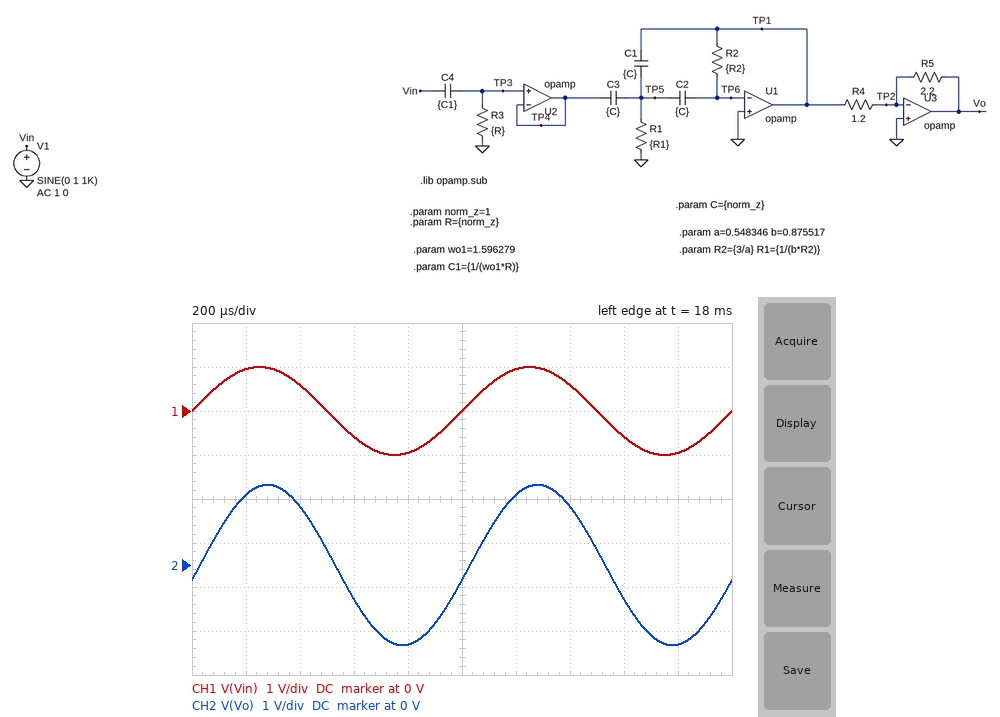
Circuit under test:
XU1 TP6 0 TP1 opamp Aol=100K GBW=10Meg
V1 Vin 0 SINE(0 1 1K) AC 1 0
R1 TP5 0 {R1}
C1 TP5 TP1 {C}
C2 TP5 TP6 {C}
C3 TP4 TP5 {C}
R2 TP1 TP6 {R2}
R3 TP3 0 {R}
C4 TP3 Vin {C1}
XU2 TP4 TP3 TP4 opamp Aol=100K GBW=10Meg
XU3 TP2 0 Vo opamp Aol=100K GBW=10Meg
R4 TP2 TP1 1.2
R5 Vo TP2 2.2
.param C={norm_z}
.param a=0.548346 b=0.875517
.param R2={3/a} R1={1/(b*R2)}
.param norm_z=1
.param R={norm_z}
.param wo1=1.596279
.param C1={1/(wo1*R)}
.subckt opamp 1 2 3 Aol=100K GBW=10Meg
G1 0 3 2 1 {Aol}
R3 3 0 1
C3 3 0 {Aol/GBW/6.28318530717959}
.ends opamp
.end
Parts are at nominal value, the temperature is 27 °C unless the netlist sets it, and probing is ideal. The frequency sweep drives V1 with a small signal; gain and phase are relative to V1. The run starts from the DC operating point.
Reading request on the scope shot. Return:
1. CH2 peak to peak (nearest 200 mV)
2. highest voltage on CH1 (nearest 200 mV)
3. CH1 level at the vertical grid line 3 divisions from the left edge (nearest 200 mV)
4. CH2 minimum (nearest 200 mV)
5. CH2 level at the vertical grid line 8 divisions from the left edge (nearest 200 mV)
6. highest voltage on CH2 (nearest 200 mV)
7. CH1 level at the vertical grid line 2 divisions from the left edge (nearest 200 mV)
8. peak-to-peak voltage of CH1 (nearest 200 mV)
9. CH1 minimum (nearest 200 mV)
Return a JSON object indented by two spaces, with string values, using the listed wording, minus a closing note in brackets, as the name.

{
  "CH2 peak to peak": "3.6 V",
  "highest voltage on CH1": "1.0 V",
  "CH1 level at the vertical grid line 3 divisions from the left edge": "-600 mV",
  "CH2 minimum": "-1.8 V",
  "CH2 level at the vertical grid line 8 divisions from the left edge": "-800 mV",
  "highest voltage on CH2": "1.8 V",
  "CH1 level at the vertical grid line 2 divisions from the left edge": "600 mV",
  "peak-to-peak voltage of CH1": "2.0 V",
  "CH1 minimum": "-1.0 V"
}
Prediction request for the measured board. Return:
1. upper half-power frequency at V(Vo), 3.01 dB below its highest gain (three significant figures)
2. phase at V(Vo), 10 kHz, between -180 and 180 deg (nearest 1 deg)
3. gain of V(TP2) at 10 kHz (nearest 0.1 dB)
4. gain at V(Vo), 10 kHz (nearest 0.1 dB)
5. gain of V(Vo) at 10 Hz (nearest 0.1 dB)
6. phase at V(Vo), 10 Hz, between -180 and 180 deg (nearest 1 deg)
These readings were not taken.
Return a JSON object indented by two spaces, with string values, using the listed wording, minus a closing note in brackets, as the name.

{
  "upper half-power frequency at V(Vo), 3.01 dB below its highest gain": "11.2 kHz",
  "phase at V(Vo), 10 kHz, between -180 and 180 deg": "-84 deg",
  "gain of V(TP2) at 10 kHz": "-57.4 dB",
  "gain at V(Vo), 10 kHz": "2.6 dB",
  "gain of V(Vo) at 10 Hz": "5.3 dB",
  "phase at V(Vo), 10 Hz, between -180 and 180 deg": "2 deg"
}
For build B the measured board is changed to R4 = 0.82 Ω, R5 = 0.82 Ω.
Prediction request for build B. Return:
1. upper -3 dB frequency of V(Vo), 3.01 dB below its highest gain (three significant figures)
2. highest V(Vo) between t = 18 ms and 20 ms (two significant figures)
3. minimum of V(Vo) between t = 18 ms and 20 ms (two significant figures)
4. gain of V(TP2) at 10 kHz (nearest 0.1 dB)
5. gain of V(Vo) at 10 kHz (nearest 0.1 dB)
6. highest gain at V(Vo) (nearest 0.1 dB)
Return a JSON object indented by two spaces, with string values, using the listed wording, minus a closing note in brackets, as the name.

{
  "upper -3 dB frequency of V(Vo), 3.01 dB below its highest gain": "11.2 kHz",
  "highest V(Vo) between t = 18 ms and 20 ms": "990 mV",
  "minimum of V(Vo) between t = 18 ms and 20 ms": "-990 mV",
  "gain of V(TP2) at 10 kHz": "-62.7 dB",
  "gain of V(Vo) at 10 kHz": "-2.7 dB",
  "highest gain at V(Vo)": "0 dB"
}
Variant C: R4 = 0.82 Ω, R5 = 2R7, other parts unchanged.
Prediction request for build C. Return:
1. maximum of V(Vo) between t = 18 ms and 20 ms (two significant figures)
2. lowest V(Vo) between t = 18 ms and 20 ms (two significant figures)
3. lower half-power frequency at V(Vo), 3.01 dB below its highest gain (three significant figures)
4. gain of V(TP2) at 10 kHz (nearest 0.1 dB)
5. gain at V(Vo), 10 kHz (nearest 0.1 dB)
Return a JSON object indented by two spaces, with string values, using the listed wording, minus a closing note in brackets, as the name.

{
  "maximum of V(Vo) between t = 18 ms and 20 ms": "3.3 V",
  "lowest V(Vo) between t = 18 ms and 20 ms": "-3.3 V",
  "lower half-power frequency at V(Vo), 3.01 dB below its highest gain": "136 mHz",
  "gain of V(TP2) at 10 kHz": "-52.3 dB",
  "gain at V(Vo), 10 kHz": "7.7 dB"
}
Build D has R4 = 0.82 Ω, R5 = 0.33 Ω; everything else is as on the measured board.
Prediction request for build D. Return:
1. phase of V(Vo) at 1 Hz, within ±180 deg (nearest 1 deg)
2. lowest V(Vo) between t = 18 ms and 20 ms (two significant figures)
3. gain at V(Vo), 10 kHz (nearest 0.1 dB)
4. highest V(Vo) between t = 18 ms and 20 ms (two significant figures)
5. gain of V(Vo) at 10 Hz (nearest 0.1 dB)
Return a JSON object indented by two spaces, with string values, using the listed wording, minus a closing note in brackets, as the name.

{
  "phase of V(Vo) at 1 Hz, within ±180 deg": "19 deg",
  "lowest V(Vo) between t = 18 ms and 20 ms": "-400 mV",
  "gain at V(Vo), 10 kHz": "-10.6 dB",
  "highest V(Vo) between t = 18 ms and 20 ms": "400 mV",
  "gain of V(Vo) at 10 Hz": "-7.9 dB"
}
